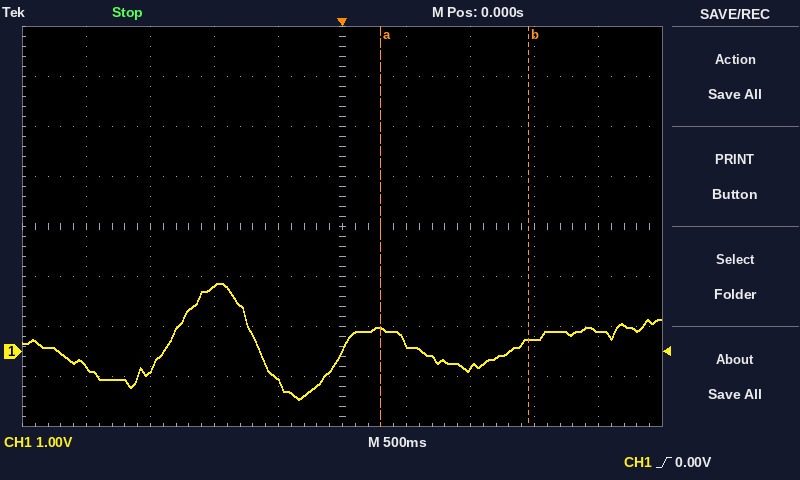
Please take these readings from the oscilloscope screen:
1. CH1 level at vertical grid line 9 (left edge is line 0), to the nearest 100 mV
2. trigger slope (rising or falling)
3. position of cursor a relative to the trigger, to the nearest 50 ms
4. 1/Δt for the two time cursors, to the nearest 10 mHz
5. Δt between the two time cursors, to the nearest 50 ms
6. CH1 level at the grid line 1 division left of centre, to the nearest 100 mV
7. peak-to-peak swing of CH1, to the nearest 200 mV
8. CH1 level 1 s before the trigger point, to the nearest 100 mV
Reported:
400 mV
rising
+300 ms
870 mHz
1.15 s
-600 mV
2.4 V
1.3 V
